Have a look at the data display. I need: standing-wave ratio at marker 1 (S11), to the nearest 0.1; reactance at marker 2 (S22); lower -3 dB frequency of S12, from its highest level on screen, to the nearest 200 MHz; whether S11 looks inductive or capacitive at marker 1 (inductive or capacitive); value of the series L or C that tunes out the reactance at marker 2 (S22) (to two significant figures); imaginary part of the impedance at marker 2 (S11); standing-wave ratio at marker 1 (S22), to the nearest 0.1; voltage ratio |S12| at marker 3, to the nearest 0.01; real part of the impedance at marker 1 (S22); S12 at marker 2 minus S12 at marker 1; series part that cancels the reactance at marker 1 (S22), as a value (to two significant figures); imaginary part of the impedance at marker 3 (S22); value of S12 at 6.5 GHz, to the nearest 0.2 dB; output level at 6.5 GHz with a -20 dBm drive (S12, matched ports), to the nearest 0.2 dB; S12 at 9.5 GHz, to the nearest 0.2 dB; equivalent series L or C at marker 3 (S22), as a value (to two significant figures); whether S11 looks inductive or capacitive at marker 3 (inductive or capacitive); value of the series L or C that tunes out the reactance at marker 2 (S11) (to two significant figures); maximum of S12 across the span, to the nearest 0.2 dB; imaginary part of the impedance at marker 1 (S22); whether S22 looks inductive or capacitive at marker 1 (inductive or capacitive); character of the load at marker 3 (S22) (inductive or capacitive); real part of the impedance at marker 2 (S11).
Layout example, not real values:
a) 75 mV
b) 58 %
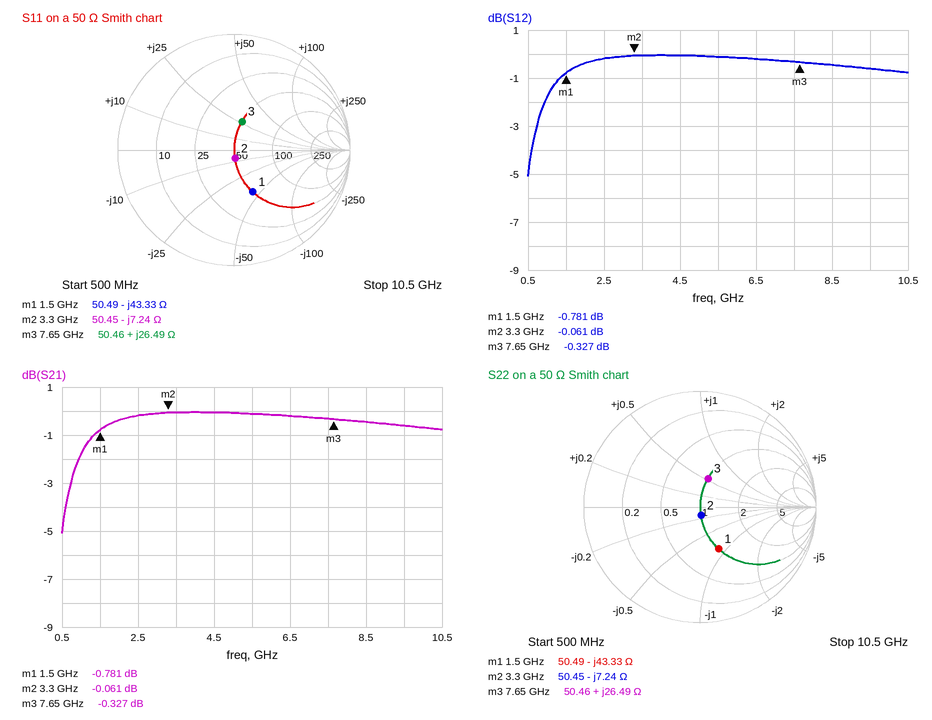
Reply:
a) 2.3
b) -7.24 Ω
c) 800 MHz
d) capacitive
e) 350 pH
f) -7.24 Ω
g) 2.3
h) 0.96
i) 50.49 Ω
j) 0.720 dB
k) 4.6 nH
l) +26.49 Ω
m) -0.2 dB
n) -20.2 dBm
o) -0.6 dB
p) 550 pH
q) inductive
r) 350 pH
s) 0.0 dB
t) -43.33 Ω
u) capacitive
v) inductive
w) 50.45 Ω
